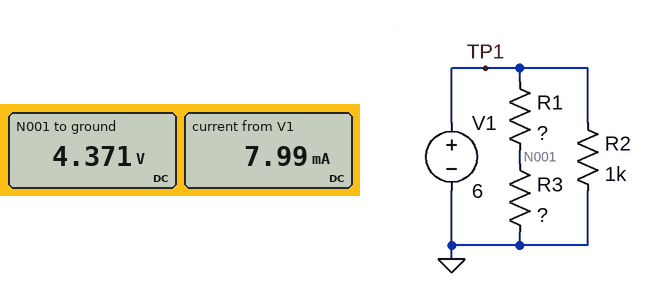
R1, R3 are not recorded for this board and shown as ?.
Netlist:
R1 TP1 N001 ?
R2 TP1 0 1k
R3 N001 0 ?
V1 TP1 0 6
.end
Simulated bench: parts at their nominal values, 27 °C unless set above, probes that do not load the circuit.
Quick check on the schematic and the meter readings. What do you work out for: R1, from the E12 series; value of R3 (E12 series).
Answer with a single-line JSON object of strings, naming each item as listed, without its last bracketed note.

{"R1, from the E12 series": "820 Ω", "value of R3": "2.2 kΩ"}
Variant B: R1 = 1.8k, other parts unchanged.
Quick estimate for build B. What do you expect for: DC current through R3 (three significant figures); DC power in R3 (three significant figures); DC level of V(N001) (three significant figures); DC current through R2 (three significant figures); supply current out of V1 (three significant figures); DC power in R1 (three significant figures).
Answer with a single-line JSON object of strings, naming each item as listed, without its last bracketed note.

{"DC current through R3": "1.50 mA", "DC power in R3": "4.95 mW", "DC level of V(N001)": "3.30 V", "DC current through R2": "6.00 mA", "supply current out of V1": "7.50 mA", "DC power in R1": "4.05 mW"}
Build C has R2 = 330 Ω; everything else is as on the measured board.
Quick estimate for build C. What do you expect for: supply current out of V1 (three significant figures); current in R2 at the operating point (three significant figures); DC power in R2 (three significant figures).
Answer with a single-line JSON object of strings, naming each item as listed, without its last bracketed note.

{"supply current out of V1": "20.2 mA", "current in R2 at the operating point": "18.2 mA", "DC power in R2": "109 mW"}
